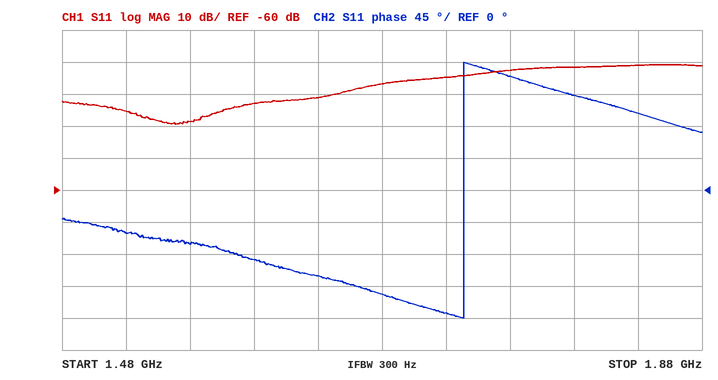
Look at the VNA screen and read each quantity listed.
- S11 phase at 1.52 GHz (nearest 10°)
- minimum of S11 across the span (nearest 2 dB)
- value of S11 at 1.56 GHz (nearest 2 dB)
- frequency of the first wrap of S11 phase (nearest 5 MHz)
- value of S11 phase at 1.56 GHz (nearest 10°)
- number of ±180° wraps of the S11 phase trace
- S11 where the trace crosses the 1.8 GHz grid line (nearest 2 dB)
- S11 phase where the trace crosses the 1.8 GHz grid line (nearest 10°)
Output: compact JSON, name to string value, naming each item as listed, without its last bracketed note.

{"S11 phase at 1.52 GHz": "-60°", "minimum of S11 across the span": "-40 dB", "value of S11 at 1.56 GHz": "-38 dB", "frequency of the first wrap of S11 phase": "1.730 GHz", "value of S11 phase at 1.56 GHz": "-80°", "number of ±180° wraps of the S11 phase trace": "1", "S11 where the trace crosses the 1.8 GHz grid line": "-22 dB", "S11 phase where the trace crosses the 1.8 GHz grid line": "130°"}
